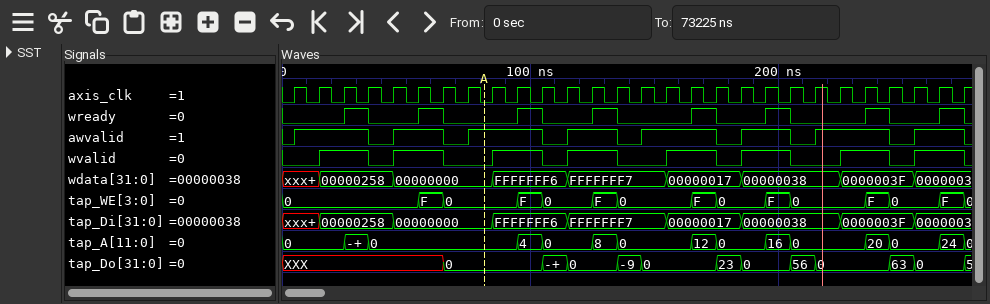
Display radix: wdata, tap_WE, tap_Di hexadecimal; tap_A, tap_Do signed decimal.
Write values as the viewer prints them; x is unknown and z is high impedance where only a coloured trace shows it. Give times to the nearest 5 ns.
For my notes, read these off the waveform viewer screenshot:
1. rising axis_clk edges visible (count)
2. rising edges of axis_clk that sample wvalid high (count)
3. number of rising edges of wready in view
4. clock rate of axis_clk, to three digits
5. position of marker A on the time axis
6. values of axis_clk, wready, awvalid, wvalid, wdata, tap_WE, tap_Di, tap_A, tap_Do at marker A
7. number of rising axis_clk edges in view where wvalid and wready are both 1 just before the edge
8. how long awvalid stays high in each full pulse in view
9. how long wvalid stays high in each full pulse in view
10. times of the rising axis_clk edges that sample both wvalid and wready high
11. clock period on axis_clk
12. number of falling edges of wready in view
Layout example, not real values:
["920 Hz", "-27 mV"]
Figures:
["28", "16", "8", "100 MHz", "80 ns", "axis_clk=0, wready=0, awvalid=1, wvalid=0, wdata=00000000, tap_WE=0, tap_Di=00000000, tap_A=0, tap_Do=0", "8", "30 ns, 20 ns, 30 ns, 20 ns, 30 ns, 20 ns, 30 ns, 20 ns", "20 ns, 20 ns, 20 ns, 20 ns, 20 ns, 20 ns, 20 ns, 20 ns", "35 ns, 65 ns, 105 ns, 135 ns, 175 ns, 205 ns, 245 ns, 275 ns", "10 ns", "8"]
